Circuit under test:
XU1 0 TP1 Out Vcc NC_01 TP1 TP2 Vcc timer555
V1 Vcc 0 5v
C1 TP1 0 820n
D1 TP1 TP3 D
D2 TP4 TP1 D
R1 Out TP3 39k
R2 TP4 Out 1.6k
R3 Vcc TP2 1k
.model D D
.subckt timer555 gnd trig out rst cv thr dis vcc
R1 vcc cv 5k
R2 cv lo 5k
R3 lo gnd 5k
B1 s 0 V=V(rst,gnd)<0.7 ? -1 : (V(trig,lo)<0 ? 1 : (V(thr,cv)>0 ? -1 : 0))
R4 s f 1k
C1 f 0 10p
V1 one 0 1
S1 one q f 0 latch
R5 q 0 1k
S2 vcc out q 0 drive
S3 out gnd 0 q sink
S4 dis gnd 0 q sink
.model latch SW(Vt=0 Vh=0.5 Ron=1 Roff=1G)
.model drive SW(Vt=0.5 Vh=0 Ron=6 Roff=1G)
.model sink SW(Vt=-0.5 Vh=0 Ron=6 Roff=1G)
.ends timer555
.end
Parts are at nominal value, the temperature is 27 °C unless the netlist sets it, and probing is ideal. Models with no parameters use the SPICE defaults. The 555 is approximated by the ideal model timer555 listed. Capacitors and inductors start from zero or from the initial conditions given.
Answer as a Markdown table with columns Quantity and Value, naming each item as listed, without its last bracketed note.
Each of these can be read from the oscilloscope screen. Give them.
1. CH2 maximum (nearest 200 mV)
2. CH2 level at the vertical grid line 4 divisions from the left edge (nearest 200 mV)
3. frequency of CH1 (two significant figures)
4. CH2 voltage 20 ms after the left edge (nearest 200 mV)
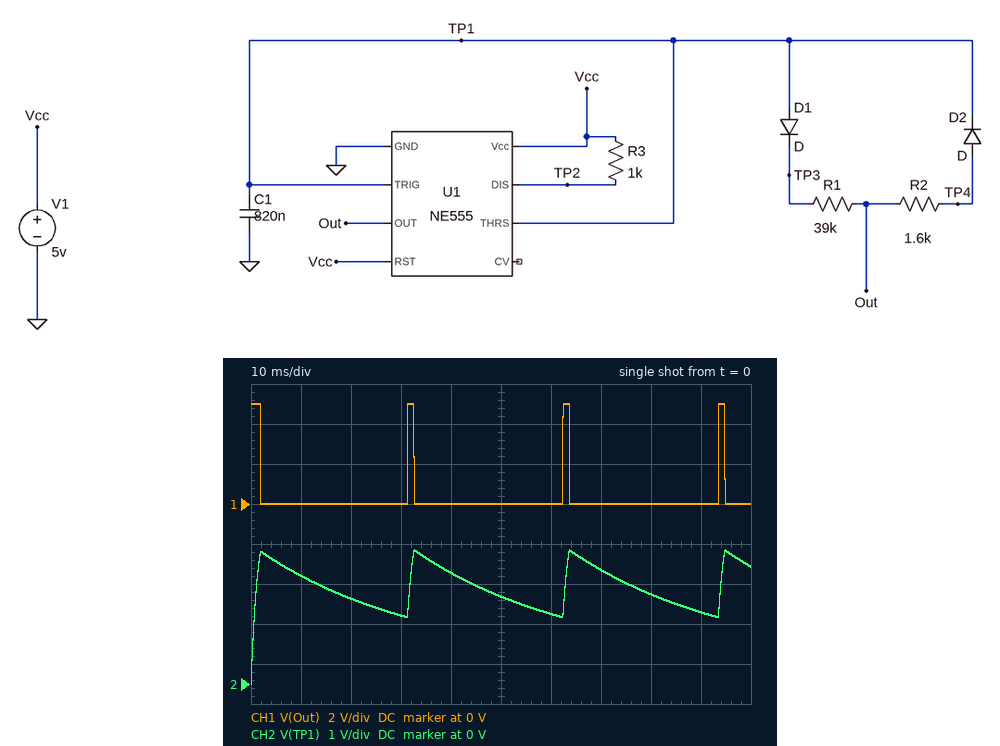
| Quantity | Value |
|---|---|
| CH2 maximum | 3.4 V |
| CH2 level at the vertical grid line 4 divisions from the left edge | 2.8 V |
| frequency of CH1 | 32 Hz |
| CH2 voltage 20 ms after the left edge | 2.2 V |
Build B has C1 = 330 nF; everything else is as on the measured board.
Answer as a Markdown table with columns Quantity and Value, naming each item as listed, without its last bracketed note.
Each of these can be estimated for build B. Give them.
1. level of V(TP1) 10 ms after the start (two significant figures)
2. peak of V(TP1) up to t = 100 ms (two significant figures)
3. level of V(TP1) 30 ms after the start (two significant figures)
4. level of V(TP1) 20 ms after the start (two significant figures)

| Quantity | Value |
|---|---|
| level of V(TP1) 10 ms after the start | 1.9 V |
| peak of V(TP1) up to t = 100 ms | 3.3 V |
| level of V(TP1) 30 ms after the start | 2.5 V |
| level of V(TP1) 20 ms after the start | 2.2 V |
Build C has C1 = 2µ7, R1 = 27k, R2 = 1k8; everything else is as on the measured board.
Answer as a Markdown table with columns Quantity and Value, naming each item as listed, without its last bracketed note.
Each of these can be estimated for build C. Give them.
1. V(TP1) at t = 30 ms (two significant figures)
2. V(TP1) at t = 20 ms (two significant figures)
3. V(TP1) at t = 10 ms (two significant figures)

| Quantity | Value |
|---|---|
| V(TP1) at t = 30 ms | 2.6 V |
| V(TP1) at t = 20 ms | 2.9 V |
| V(TP1) at t = 10 ms | 3.2 V |
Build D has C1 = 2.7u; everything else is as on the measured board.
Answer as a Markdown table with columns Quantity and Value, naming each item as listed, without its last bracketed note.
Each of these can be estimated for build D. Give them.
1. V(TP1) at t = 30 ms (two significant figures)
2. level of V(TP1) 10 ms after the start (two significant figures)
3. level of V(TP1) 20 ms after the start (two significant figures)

| Quantity | Value |
|---|---|
| V(TP1) at t = 30 ms | 2.8 V |
| level of V(TP1) 10 ms after the start | 3.2 V |
| level of V(TP1) 20 ms after the start | 3.0 V |
